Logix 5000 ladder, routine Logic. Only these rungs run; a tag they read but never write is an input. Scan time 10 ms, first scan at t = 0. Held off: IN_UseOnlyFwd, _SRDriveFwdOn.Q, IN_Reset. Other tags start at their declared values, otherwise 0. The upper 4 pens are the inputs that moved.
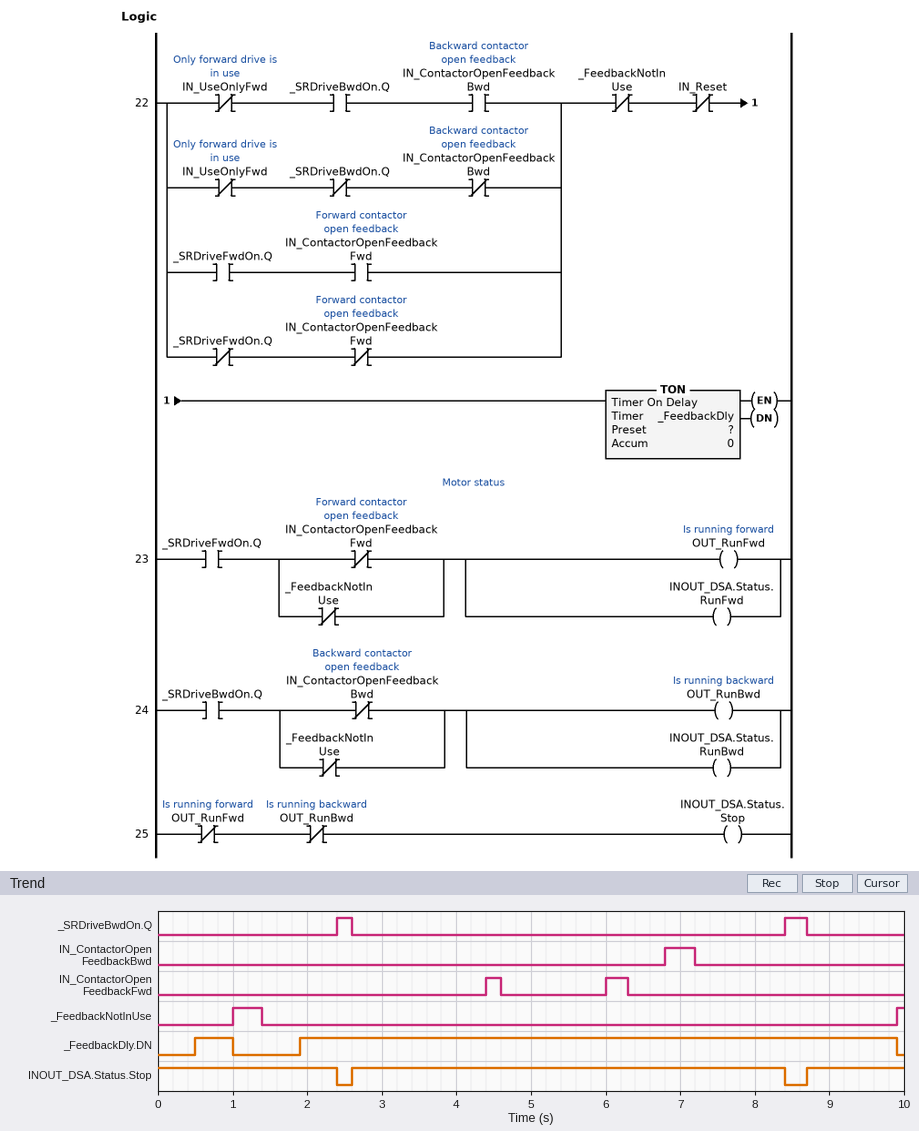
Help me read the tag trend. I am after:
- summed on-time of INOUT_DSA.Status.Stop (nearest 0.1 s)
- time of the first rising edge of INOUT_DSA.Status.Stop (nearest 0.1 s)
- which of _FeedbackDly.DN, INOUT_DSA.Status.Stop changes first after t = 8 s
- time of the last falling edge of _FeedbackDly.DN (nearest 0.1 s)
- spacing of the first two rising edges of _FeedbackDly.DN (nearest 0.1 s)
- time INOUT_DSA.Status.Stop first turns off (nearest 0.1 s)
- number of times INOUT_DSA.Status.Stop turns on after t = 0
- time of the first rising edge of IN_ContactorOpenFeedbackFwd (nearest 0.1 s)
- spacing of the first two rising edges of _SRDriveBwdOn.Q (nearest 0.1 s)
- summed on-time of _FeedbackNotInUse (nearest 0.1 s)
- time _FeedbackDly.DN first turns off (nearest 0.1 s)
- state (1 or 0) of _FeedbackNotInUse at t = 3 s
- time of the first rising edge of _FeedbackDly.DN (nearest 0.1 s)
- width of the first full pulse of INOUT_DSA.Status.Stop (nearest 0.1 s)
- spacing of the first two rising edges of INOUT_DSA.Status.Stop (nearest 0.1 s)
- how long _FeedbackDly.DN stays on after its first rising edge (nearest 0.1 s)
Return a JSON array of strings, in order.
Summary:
["9.5 s", "2.6 s", "INOUT_DSA.Status.Stop", "9.9 s", "1.4 s", "2.4 s", "2", "4.4 s", "6.0 s", "0.5 s", "1.0 s", "0", "0.5 s", "5.8 s", "6.1 s", "0.5 s"]
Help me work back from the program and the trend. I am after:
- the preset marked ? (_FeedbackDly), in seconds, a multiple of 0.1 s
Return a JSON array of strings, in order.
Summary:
["0.5 s"]
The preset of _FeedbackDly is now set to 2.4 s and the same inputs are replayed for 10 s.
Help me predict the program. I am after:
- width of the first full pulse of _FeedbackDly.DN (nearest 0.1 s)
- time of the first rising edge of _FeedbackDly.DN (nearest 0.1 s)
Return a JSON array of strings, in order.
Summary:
["6.1 s", "3.8 s"]
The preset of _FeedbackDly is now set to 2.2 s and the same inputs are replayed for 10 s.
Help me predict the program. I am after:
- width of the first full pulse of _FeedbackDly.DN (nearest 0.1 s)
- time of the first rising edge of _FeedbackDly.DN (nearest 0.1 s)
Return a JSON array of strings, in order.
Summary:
["6.3 s", "3.6 s"]
